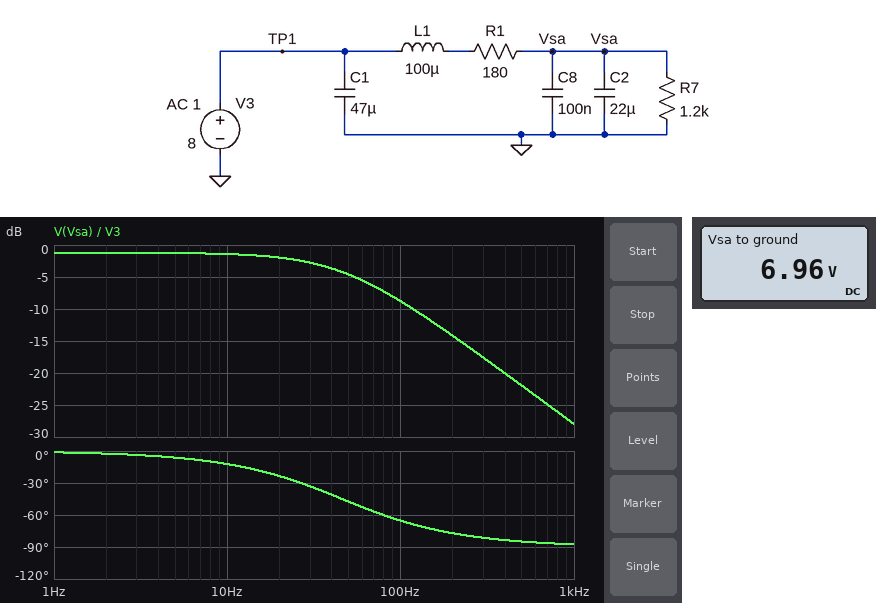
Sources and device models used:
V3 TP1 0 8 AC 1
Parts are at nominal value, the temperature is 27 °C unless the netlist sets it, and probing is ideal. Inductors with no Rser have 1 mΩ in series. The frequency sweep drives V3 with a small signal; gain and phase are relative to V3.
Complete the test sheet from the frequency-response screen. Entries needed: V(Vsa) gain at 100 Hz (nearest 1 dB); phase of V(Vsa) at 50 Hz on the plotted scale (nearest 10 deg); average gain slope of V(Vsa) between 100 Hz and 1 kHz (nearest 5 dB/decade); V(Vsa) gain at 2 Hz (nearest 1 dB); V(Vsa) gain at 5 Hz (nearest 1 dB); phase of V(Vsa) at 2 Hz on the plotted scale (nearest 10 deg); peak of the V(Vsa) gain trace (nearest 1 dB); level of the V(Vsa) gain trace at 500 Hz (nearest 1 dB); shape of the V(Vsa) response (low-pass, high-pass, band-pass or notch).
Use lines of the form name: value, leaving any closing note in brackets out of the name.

V(Vsa) gain at 100 Hz: -9 dB
phase of V(Vsa) at 50 Hz on the plotted scale: -50 deg
average gain slope of V(Vsa) between 100 Hz and 1 kHz: -20 dB/decade
V(Vsa) gain at 2 Hz: -1 dB
V(Vsa) gain at 5 Hz: -1 dB
phase of V(Vsa) at 2 Hz on the plotted scale: 0 deg
peak of the V(Vsa) gain trace: -1 dB
level of the V(Vsa) gain trace at 500 Hz: -22 dB
shape of the V(Vsa) response: low-pass
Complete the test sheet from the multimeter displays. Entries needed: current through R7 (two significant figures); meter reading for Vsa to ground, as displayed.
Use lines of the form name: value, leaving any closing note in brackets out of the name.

current through R7: 5.8 mA
meter reading for Vsa to ground, as displayed: 6.96 V
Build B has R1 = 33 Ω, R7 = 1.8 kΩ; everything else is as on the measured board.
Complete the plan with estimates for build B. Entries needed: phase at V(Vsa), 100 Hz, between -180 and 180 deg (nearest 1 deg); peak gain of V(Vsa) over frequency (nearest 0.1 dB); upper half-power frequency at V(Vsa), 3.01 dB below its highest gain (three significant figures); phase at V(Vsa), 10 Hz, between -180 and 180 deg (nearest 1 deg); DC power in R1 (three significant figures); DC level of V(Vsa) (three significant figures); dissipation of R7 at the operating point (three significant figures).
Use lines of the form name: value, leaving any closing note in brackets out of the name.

phase at V(Vsa), 100 Hz, between -180 and 180 deg: -24 deg
peak gain of V(Vsa) over frequency: -0.2 dB
upper half-power frequency at V(Vsa), 3.01 dB below its highest gain: 223 Hz
phase at V(Vsa), 10 Hz, between -180 and 180 deg: -3 deg
DC power in R1: 629 µW
DC level of V(Vsa): 7.86 V
dissipation of R7 at the operating point: 34.3 mW
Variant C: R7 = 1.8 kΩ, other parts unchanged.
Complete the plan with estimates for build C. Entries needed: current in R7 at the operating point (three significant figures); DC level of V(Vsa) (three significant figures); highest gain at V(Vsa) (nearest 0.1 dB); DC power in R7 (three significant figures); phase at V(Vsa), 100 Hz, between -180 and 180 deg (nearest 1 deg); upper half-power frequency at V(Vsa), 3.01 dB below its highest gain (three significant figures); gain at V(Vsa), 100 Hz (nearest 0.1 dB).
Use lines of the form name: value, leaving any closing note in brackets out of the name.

current in R7 at the operating point: 4.04 mA
DC level of V(Vsa): 7.27 V
highest gain at V(Vsa): -0.8 dB
DC power in R7: 29.4 mW
phase at V(Vsa), 100 Hz, between -180 and 180 deg: -66 deg
upper half-power frequency at V(Vsa), 3.01 dB below its highest gain: 44.0 Hz
gain at V(Vsa), 100 Hz: -8.7 dB
